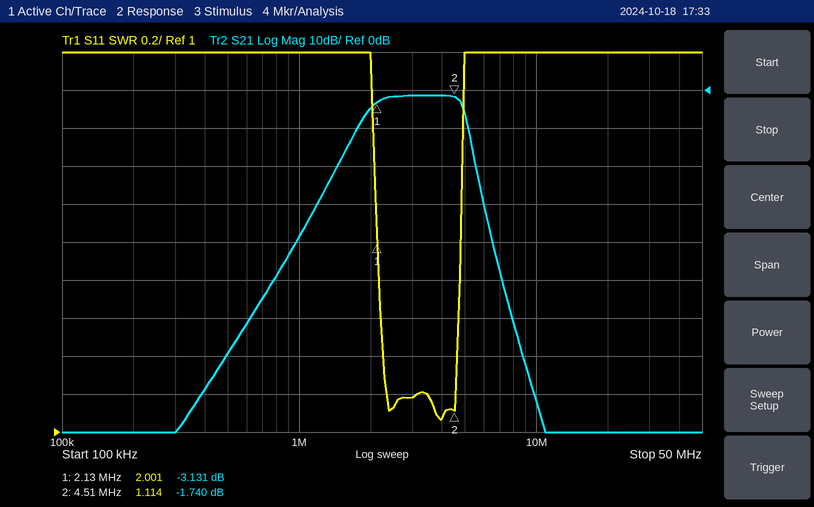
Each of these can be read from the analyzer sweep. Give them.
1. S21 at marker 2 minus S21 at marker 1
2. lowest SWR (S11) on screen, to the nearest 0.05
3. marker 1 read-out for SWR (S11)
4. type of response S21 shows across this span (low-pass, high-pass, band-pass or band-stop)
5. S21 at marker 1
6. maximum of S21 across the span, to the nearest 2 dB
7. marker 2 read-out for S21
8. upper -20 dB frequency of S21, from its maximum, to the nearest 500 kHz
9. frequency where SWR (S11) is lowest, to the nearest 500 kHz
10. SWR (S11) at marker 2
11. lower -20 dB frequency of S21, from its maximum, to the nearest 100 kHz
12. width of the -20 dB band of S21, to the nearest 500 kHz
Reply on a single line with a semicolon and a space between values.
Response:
1.391 dB; 1.05; 2.001; band-pass; -3.131 dB; -2 dB; -1.740 dB; 5.5 MHz; 4.0 MHz; 1.114; 1.4 MHz; 4.0 MHz
